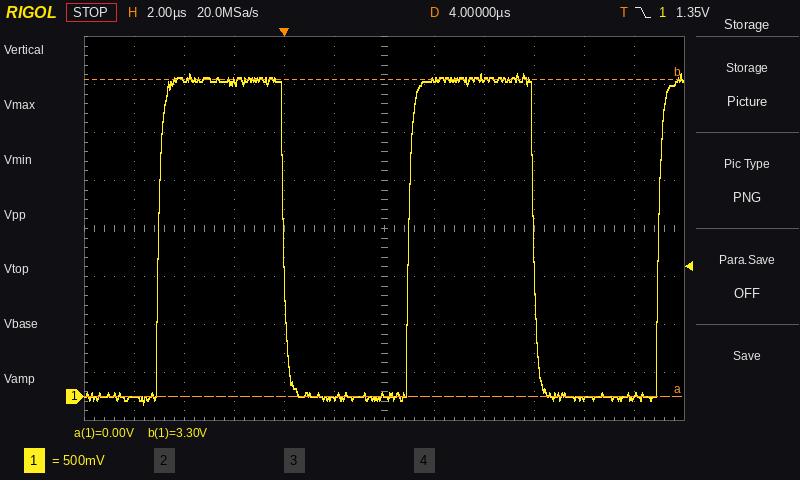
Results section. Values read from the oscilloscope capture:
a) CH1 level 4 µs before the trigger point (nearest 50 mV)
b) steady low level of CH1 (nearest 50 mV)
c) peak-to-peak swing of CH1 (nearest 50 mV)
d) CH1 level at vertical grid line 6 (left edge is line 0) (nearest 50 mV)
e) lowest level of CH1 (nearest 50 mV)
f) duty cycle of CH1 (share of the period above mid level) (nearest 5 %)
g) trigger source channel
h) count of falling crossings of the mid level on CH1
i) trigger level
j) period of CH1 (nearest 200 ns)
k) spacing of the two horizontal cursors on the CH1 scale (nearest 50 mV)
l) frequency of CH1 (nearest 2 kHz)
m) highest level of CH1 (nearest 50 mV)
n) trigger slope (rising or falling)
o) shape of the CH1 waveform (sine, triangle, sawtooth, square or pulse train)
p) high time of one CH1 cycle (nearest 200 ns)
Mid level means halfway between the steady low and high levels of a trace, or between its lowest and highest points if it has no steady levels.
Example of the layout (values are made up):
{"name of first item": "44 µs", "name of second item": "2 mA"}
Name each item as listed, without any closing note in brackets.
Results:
{"CH1 level 4 µs before the trigger point": "3.30 V", "steady low level of CH1": "0 mV", "peak-to-peak swing of CH1": "3.45 V", "CH1 level at vertical grid line 6 (left edge is line 0)": "0 mV", "lowest level of CH1": "-100 mV", "duty cycle of CH1 (share of the period above mid level)": "50 %", "trigger source channel": "CH1", "count of falling crossings of the mid level on CH1": "2", "trigger level": "1.35 V", "period of CH1": "10.0 µs", "spacing of the two horizontal cursors on the CH1 scale": "3.30 V", "frequency of CH1": "100 kHz", "highest level of CH1": "3.35 V", "trigger slope": "falling", "shape of the CH1 waveform": "square", "high time of one CH1 cycle": "5.0 µs"}
